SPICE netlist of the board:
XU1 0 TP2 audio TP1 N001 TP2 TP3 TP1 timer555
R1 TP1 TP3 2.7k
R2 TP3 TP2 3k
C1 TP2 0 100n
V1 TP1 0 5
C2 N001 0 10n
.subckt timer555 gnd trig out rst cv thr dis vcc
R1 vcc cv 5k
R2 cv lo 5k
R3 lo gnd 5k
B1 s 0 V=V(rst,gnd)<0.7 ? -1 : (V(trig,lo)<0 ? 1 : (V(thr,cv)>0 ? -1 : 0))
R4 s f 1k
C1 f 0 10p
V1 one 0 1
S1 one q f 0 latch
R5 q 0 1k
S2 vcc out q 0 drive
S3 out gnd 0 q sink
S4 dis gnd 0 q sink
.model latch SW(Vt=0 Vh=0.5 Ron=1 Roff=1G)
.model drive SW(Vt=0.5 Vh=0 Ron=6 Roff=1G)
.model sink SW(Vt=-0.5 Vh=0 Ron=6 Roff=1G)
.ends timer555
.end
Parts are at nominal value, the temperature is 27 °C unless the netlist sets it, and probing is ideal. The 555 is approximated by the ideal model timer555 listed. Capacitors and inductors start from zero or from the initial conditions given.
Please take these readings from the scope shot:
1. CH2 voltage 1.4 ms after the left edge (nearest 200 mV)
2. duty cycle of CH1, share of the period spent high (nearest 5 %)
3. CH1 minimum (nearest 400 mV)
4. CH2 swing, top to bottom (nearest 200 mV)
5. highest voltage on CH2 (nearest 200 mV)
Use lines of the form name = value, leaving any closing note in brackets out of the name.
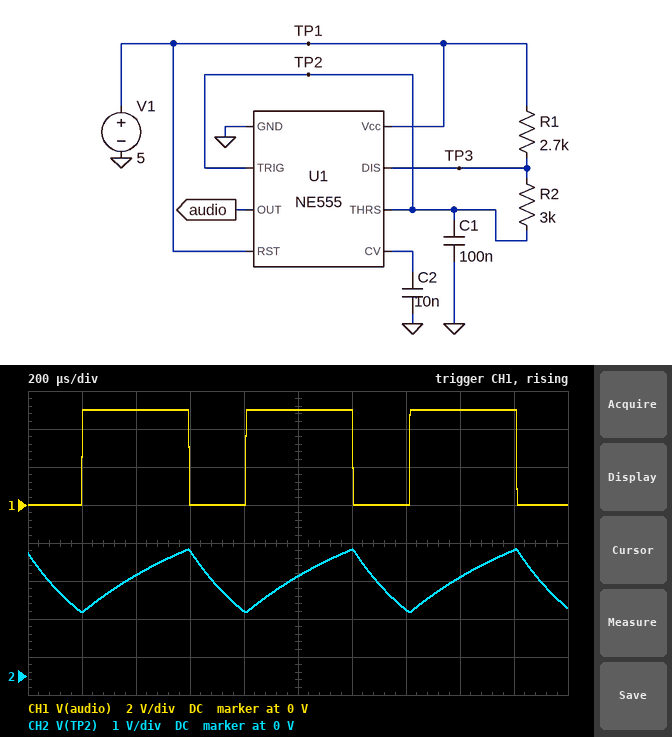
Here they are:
CH2 voltage 1.4 ms after the left edge = 1.8 V
duty cycle of CH1, share of the period spent high = 65 %
CH1 minimum = 0 V
CH2 swing, top to bottom = 1.6 V
highest voltage on CH2 = 3.4 V
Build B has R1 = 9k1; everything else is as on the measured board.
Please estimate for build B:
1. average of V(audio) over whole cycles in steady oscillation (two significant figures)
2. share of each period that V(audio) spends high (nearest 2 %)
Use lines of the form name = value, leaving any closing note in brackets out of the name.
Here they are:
average of V(audio) over whole cycles in steady oscillation = 4.0 V
share of each period that V(audio) spends high = 80 %
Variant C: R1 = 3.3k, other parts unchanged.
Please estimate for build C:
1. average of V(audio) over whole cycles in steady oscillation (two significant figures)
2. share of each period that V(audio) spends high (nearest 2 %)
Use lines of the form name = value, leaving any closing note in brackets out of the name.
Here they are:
average of V(audio) over whole cycles in steady oscillation = 3.4 V
share of each period that V(audio) spends high = 68 %
